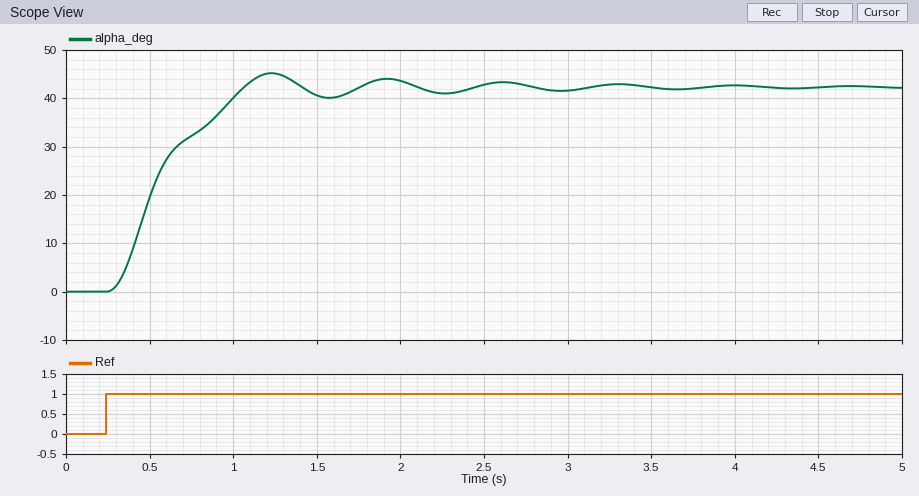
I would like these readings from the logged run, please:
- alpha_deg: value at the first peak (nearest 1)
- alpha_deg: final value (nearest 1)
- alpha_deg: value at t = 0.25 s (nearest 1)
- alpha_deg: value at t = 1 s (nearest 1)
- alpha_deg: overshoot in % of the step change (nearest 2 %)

45
42
0
40
6 %
